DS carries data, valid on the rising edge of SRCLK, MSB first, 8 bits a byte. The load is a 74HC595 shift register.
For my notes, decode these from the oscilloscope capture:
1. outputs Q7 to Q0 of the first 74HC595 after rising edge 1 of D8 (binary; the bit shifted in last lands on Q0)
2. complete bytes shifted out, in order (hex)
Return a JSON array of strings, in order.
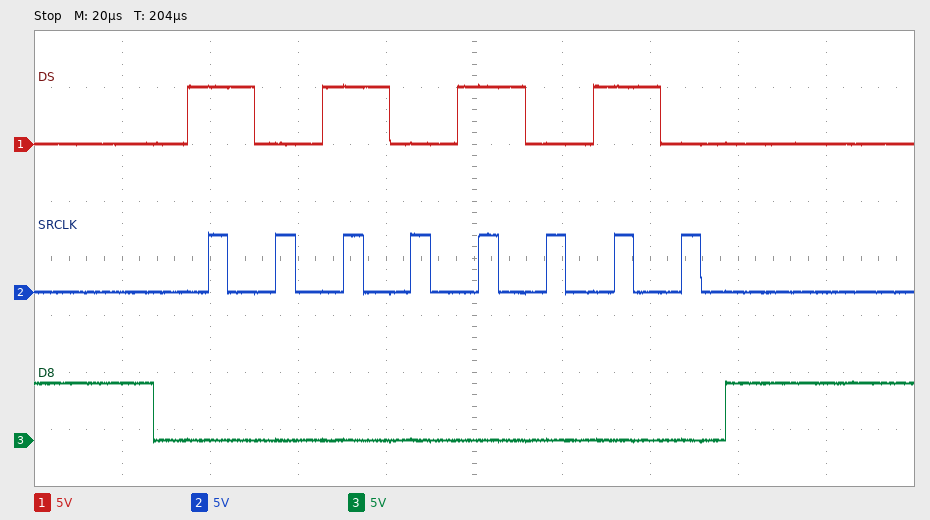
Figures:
["10101010", "AA"]
